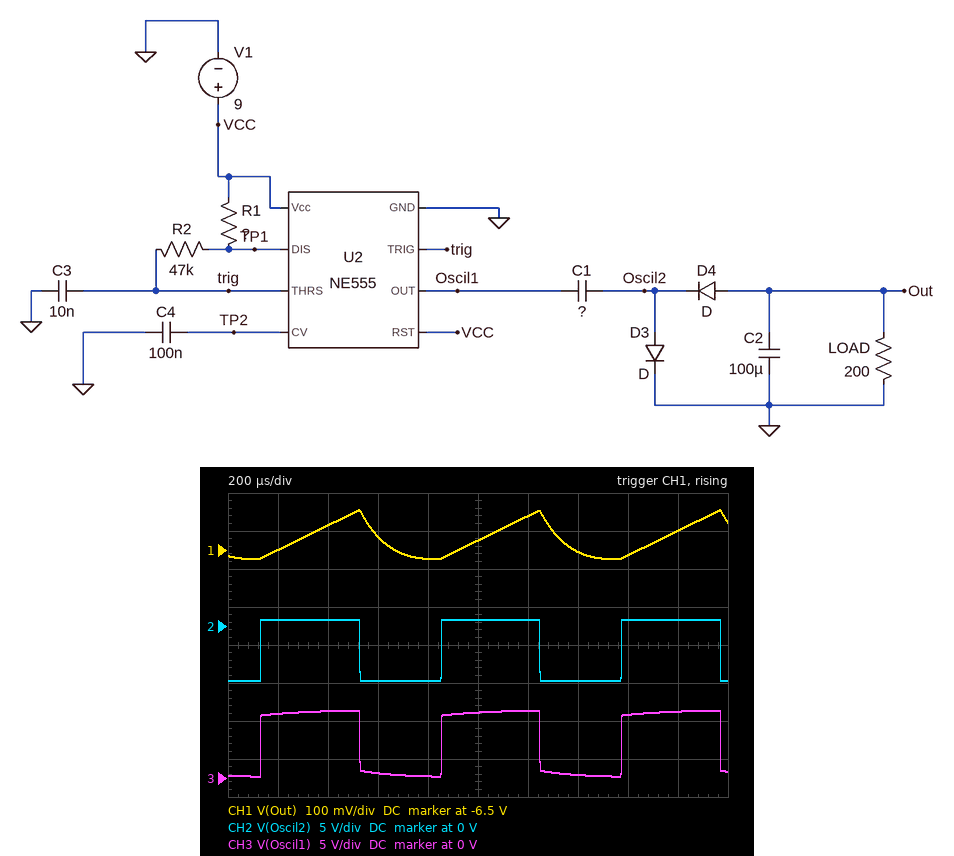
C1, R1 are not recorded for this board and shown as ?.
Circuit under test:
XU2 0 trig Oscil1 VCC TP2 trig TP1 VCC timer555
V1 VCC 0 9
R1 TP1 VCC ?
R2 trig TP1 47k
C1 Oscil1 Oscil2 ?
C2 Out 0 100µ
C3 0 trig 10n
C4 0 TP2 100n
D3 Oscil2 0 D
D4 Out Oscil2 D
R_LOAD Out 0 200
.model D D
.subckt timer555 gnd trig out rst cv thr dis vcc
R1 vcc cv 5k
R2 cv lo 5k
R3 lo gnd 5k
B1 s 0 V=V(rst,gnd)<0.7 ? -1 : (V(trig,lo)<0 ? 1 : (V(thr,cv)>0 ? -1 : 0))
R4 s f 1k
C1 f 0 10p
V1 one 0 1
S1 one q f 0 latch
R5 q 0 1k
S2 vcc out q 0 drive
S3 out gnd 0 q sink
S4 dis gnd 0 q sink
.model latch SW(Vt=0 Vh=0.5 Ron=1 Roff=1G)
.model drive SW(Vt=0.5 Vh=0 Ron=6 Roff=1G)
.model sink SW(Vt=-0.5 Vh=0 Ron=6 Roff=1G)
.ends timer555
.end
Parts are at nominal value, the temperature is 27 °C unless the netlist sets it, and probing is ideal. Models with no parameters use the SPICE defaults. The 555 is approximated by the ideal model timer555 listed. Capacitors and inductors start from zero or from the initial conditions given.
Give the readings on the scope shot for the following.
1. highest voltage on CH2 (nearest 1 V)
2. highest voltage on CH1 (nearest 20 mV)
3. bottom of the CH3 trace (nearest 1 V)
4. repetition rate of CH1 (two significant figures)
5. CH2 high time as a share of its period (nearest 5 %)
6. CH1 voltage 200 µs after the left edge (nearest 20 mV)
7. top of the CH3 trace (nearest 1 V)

1 V
-6.40 V
0 V
1.4 kHz
55 %
-6.50 V
9 V
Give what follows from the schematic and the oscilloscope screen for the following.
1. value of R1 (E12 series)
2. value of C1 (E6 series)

10 kΩ
33 µF
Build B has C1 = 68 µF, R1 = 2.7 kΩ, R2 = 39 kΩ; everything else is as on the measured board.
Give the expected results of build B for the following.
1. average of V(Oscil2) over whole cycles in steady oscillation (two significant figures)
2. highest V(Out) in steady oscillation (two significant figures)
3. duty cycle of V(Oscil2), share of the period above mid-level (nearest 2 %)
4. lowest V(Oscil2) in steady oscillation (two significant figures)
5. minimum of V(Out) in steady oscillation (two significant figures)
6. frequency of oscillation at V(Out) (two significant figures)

-3.2 V
-6.6 V
52 %
-7.4 V
-6.7 V
1.8 kHz
